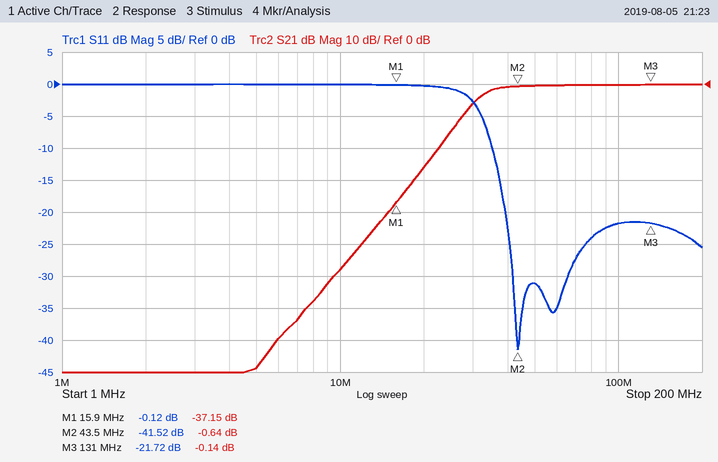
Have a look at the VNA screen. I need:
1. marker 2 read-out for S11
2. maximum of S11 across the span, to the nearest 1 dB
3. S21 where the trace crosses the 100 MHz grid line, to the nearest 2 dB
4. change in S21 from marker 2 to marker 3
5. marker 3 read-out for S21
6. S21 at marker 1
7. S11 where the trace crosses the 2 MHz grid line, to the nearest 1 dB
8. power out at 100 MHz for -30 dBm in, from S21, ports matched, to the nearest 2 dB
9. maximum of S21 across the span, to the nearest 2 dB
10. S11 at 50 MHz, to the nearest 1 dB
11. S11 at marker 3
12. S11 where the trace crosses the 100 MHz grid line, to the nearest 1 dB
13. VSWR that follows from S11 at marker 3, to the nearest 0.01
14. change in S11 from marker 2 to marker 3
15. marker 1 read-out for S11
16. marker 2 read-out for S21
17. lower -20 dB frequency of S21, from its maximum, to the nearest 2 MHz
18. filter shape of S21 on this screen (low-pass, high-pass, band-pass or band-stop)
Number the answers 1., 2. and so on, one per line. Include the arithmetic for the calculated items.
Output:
1. -41.52 dB
2. 0 dB
3. 0 dB
4. -0.14 − (-0.64) = 0.50 dB
5. -0.14 dB
6. -37.15 dB
7. 0 dB
8. -30 dBm + (0 dB) = -30 dBm
9. 0 dB
10. -31 dB
11. -21.72 dB
12. -22 dB
13. (1 + 0.0820)/(1 − 0.0820) ≈ 1.18
14. -21.72 − (-41.52) = 19.80 dB
15. -0.12 dB
16. -0.64 dB
17. 22 MHz
18. high-pass
